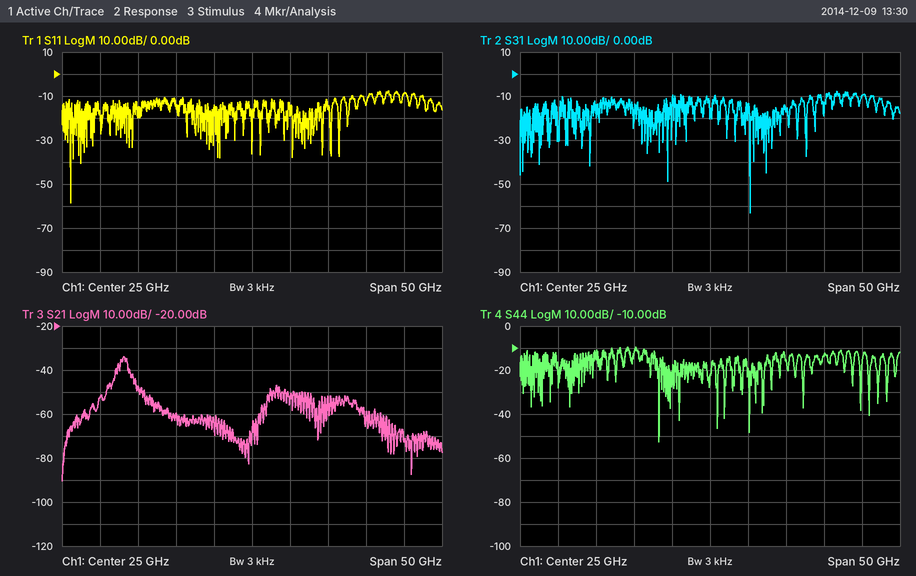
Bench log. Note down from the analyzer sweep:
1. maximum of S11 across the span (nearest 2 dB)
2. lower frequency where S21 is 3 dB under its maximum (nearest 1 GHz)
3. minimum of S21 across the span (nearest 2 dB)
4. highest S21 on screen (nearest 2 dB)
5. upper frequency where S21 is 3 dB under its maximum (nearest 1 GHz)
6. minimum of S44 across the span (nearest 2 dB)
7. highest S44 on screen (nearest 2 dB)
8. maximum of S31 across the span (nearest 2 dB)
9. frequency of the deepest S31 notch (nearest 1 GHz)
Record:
-8 dB
8 GHz
-90 dB
-34 dB
9 GHz
-52 dB
-10 dB
-8 dB
30 GHz
